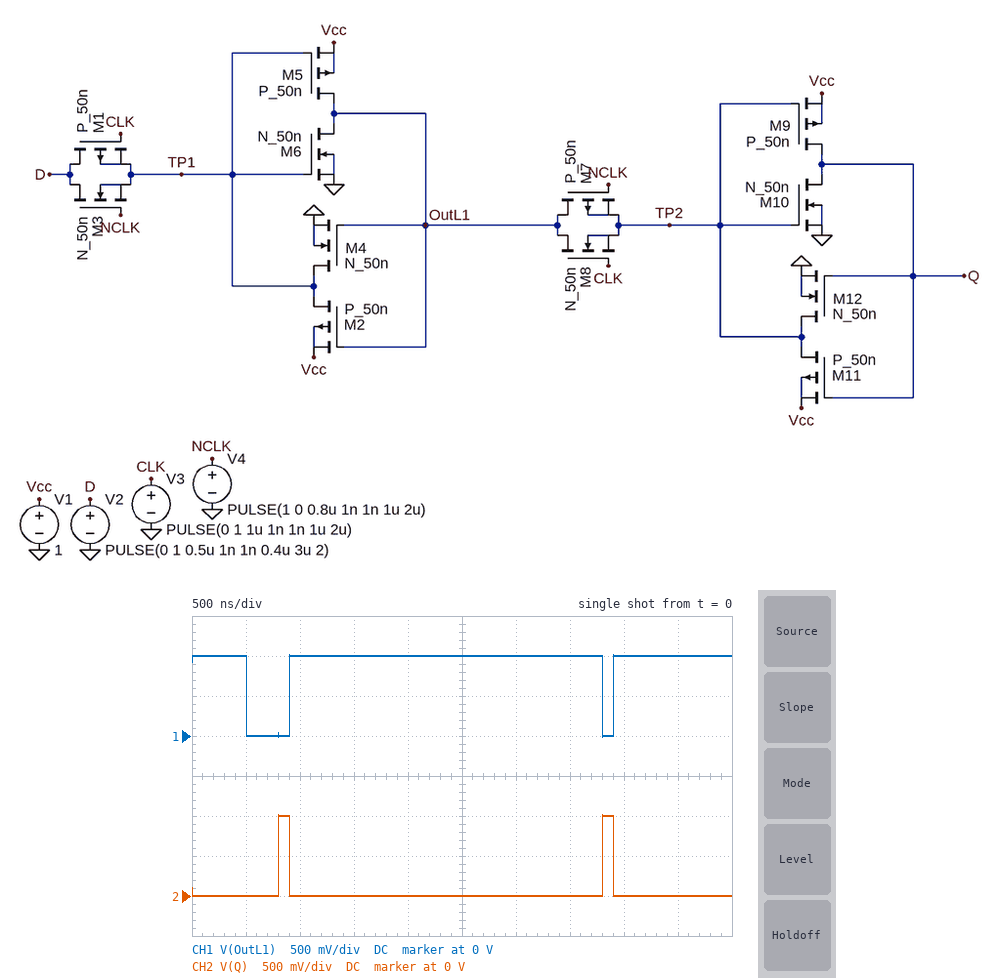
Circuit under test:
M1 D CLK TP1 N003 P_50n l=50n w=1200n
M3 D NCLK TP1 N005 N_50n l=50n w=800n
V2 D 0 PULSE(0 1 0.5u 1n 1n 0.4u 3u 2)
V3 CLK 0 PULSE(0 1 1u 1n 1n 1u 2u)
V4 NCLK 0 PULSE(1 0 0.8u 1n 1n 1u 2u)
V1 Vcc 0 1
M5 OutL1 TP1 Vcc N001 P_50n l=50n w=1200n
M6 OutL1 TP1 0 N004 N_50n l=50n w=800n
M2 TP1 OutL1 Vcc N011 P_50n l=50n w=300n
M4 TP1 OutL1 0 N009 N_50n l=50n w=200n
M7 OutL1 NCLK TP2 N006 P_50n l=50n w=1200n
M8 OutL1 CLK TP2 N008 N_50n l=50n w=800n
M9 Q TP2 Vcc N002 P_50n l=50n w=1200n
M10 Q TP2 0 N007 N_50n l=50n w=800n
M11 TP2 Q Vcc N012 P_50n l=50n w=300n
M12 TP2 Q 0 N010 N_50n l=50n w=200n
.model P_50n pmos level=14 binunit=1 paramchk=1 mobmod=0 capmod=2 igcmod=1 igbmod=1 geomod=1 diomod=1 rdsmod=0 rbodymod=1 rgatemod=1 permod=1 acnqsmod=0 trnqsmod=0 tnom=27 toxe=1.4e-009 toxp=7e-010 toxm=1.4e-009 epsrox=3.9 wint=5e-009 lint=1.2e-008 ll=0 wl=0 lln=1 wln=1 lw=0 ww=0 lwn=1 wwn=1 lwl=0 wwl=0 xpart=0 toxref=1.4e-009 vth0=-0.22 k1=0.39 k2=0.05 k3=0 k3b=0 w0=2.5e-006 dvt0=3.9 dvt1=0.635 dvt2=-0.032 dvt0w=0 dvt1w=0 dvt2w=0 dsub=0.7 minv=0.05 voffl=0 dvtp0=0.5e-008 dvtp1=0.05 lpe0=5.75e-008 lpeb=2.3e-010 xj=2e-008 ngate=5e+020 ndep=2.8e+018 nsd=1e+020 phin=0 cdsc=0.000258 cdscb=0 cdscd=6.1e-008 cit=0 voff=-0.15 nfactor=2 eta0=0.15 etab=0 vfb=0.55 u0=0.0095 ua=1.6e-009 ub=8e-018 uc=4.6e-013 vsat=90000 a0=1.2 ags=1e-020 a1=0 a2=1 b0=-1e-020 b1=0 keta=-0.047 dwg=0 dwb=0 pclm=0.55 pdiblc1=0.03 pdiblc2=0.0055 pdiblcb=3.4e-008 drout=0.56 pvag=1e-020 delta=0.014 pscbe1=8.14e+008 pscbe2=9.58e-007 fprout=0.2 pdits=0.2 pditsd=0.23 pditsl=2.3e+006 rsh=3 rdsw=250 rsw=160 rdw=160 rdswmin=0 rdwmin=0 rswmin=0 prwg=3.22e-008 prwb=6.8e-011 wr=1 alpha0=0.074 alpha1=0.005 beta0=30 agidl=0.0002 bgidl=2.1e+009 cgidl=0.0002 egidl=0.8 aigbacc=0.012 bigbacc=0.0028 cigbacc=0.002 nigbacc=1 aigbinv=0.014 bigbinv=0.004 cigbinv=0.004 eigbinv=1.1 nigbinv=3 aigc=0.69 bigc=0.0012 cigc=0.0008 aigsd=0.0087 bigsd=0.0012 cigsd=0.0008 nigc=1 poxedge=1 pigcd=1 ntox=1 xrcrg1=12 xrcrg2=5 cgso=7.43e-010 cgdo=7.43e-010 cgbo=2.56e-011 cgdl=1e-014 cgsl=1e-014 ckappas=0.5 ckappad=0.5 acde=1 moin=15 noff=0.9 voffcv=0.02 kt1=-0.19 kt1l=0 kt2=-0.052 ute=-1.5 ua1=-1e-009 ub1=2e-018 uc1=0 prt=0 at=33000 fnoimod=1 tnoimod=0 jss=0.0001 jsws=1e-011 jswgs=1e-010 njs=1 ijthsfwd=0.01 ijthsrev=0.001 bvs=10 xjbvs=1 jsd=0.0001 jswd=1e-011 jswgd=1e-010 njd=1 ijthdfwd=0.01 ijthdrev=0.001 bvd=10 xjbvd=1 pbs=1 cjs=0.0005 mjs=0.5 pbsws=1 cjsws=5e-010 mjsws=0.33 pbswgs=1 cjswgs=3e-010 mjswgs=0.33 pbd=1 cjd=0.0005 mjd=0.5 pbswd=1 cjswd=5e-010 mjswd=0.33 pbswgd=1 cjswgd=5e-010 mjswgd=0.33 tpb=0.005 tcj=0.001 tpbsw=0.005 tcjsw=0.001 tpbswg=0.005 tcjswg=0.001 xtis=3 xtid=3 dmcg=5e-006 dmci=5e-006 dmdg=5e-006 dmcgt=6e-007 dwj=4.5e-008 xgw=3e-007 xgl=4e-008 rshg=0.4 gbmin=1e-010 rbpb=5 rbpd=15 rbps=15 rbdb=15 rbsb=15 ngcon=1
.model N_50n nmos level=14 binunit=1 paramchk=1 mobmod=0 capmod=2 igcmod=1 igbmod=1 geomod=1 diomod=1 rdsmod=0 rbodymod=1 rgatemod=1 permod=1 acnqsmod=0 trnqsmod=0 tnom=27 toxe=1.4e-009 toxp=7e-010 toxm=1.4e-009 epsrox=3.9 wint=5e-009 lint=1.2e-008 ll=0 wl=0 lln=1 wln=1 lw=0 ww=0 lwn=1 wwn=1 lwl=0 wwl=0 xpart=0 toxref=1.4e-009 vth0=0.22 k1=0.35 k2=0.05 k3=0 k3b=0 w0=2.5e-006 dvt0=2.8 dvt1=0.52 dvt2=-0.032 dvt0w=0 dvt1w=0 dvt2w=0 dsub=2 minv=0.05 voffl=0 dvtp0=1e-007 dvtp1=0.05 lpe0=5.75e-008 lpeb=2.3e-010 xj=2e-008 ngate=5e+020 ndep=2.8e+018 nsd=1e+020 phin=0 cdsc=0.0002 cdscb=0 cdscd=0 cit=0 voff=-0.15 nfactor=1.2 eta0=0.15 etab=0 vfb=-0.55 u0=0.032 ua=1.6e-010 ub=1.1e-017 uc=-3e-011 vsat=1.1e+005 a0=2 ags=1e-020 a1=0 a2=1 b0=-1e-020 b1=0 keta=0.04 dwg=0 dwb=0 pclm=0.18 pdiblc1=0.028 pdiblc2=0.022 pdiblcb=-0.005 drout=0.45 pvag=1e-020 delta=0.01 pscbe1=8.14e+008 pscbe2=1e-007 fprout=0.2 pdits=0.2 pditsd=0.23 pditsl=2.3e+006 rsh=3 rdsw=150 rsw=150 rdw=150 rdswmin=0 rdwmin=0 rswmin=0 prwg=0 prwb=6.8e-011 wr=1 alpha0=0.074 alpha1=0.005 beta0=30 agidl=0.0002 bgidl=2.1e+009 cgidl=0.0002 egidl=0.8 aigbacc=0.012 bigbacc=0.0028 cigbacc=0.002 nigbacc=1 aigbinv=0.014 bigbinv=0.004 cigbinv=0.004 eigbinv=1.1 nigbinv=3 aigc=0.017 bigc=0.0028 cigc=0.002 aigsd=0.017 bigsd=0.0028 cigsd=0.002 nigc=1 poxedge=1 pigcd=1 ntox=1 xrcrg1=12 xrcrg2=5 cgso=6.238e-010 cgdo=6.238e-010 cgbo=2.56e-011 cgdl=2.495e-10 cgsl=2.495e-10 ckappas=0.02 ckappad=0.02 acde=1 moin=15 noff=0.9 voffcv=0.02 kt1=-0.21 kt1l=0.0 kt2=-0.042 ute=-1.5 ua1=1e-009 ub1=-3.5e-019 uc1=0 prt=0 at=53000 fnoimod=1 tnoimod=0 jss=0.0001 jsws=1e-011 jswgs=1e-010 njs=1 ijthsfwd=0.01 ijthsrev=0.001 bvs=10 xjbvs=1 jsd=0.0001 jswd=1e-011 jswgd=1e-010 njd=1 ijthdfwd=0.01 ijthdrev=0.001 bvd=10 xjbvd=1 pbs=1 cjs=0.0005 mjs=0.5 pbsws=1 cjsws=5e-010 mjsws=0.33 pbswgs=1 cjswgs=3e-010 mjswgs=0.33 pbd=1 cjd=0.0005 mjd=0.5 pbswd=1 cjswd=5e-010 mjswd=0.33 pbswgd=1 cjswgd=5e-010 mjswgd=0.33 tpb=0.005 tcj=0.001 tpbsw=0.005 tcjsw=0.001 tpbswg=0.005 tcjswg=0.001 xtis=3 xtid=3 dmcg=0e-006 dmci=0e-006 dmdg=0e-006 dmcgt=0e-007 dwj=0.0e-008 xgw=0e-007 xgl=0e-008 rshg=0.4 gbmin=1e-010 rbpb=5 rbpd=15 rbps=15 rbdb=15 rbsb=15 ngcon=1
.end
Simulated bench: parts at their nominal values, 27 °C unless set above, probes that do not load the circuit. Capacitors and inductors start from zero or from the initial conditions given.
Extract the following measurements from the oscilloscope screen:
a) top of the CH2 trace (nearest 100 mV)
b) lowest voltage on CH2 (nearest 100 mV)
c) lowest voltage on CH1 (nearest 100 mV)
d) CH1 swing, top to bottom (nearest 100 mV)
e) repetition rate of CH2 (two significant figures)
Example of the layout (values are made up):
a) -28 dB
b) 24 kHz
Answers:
a) 1.0 V
b) 0 V
c) 0 V
d) 1.0 V
e) 330 kHz
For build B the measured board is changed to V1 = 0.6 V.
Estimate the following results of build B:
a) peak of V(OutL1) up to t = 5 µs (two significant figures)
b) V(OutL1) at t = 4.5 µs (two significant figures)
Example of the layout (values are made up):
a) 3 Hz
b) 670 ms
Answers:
a) 610 mV
b) 600 mV
